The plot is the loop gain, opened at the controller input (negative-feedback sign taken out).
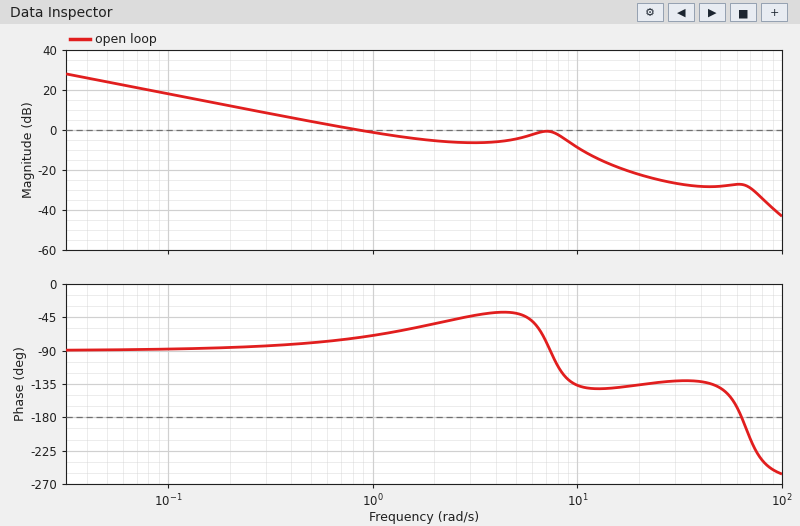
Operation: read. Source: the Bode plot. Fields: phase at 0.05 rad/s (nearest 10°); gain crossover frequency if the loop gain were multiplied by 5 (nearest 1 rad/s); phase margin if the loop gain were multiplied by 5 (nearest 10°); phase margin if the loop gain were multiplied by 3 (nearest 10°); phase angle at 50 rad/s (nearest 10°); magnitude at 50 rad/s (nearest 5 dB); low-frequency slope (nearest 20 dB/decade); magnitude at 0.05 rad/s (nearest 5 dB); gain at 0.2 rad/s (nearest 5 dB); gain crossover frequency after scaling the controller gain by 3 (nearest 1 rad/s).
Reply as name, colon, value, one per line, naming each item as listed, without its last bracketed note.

phase at 0.05 rad/s: -90°
gain crossover frequency if the loop gain were multiplied by 5: 12 rad/s
phase margin if the loop gain were multiplied by 5: 40°
phase margin if the loop gain were multiplied by 3: 40°
phase angle at 50 rad/s: -140°
magnitude at 50 rad/s: -30 dB
low-frequency slope: -20 dB/decade
magnitude at 0.05 rad/s: 25 dB
gain at 0.2 rad/s: 10 dB
gain crossover frequency after scaling the controller gain by 3: 10 rad/s
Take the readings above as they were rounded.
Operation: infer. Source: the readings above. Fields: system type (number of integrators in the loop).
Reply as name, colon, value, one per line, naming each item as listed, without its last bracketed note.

system type: 1
